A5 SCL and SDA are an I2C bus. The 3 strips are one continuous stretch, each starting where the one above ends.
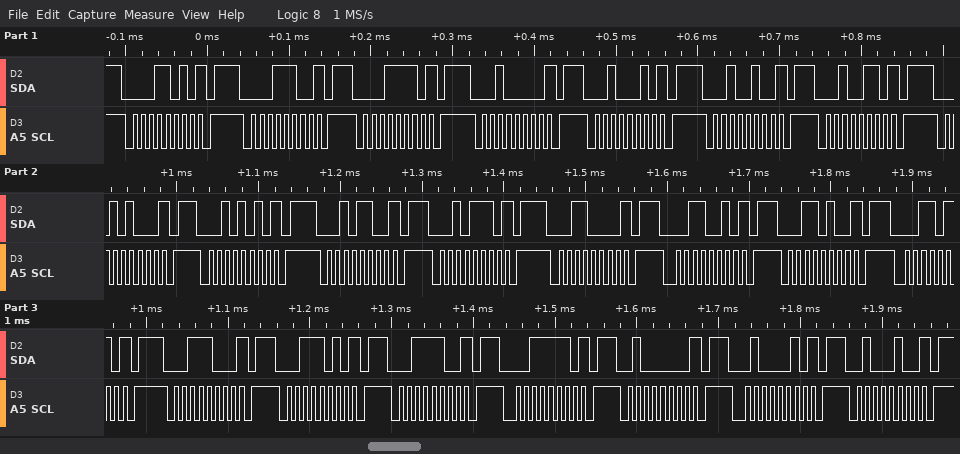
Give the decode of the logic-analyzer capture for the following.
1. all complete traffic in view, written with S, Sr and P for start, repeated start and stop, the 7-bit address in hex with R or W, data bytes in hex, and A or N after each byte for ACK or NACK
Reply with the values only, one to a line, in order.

S 0DW N P S 0EW N P S 0FW N P S 10W N P S 11W N P S 12W N P S 13W N P S 14W N P S 15W N P S 16W N P S 17W N P S 18W N P S 19W N P S 1AW N P S 1BW N P S 1CW N P S 1DW N P S 1EW N P S 1FW N P S 20W N P S 21W N P S 22W N P
